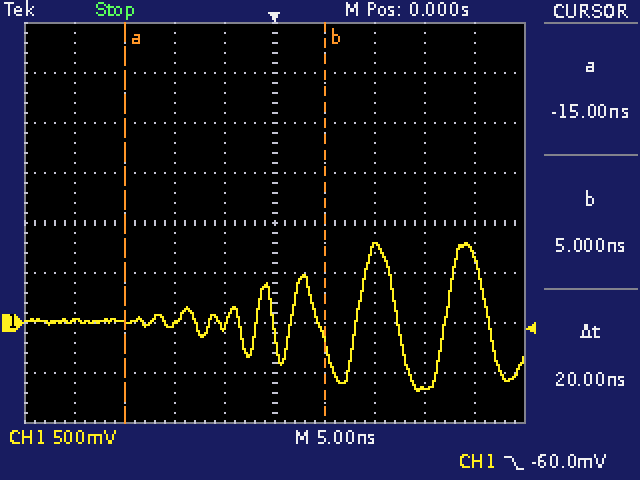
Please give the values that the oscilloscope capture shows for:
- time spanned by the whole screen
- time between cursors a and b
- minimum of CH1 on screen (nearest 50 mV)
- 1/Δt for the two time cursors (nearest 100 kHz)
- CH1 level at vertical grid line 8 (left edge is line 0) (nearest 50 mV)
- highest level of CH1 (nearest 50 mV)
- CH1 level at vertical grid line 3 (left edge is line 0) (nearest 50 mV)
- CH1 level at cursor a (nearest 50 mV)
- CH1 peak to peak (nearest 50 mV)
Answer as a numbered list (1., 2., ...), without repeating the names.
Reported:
1. 50 ns
2. 20 ns
3. -700 mV
4. 50.0 MHz
5. -650 mV
6. 800 mV
7. 0 mV
8. 0 mV
9. 1.50 V
